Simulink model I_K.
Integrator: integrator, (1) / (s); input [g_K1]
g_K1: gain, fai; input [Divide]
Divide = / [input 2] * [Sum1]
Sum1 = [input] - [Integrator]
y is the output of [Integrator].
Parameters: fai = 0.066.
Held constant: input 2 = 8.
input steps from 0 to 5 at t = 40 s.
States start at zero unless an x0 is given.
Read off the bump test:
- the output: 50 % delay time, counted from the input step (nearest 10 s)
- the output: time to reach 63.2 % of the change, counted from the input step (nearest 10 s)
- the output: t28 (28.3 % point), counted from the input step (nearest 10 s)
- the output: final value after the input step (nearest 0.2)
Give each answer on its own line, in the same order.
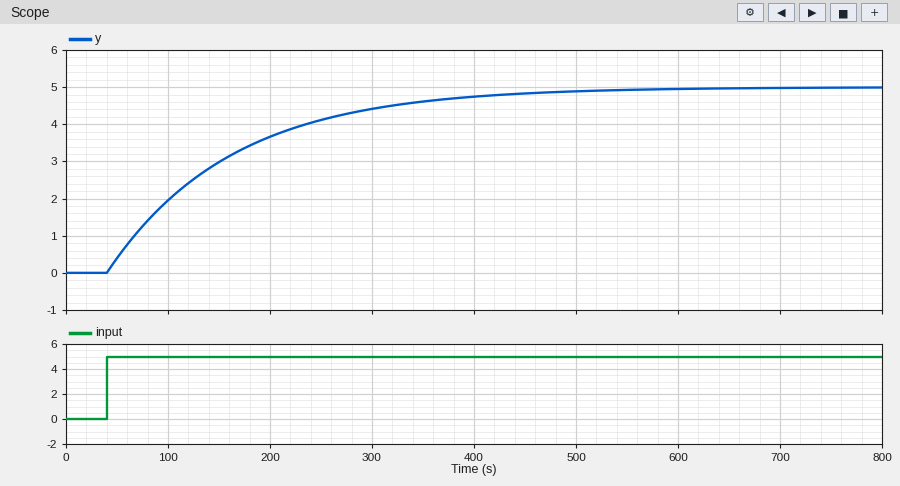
80 s
120 s
40 s
5.0
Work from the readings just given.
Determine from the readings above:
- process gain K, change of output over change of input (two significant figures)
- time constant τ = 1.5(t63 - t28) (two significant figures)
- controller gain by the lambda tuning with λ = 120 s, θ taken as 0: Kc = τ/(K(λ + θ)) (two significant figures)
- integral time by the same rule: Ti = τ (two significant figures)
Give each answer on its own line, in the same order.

1.0
120 s
1.0
120 s
